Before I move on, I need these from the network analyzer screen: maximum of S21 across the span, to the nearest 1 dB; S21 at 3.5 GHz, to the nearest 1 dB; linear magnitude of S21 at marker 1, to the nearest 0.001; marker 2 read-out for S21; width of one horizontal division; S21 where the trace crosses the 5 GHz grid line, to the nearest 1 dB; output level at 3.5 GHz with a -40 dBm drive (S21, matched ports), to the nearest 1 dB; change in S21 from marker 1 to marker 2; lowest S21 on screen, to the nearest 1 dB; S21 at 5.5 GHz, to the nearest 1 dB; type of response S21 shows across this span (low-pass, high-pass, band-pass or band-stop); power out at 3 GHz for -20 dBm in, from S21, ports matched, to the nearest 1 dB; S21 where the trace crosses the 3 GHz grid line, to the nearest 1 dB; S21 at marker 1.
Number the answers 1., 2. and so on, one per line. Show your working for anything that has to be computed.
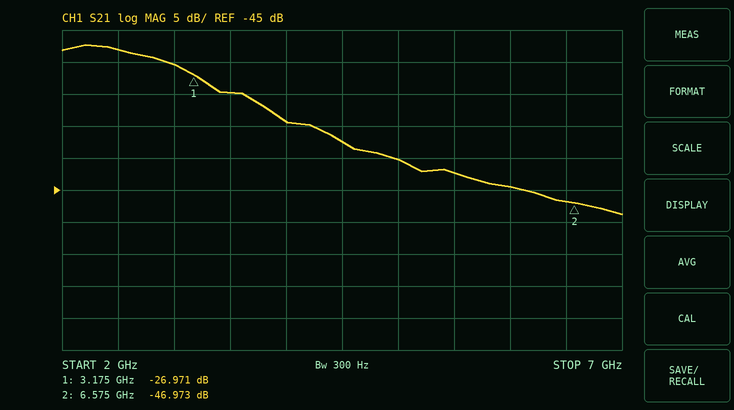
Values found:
1. -22 dB
2. -30 dB
3. 10^(-26.971/20) ≈ 0.045
4. -46.973 dB
5. 500 MHz
6. -40 dB
7. -40 dBm + (-30 dB) = -70 dBm
8. -46.973 − (-26.971) = -20.002 dB
9. -49 dB
10. -42 dB
11. low-pass
12. -20 dBm + (-25 dB) = -45 dBm
13. -25 dB
14. -26.971 dB
